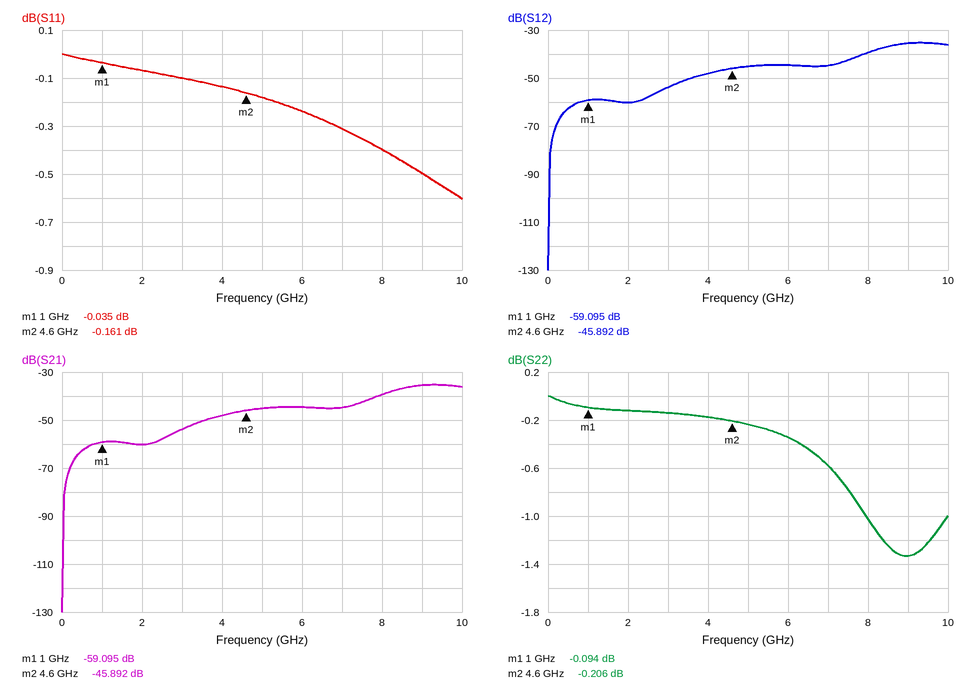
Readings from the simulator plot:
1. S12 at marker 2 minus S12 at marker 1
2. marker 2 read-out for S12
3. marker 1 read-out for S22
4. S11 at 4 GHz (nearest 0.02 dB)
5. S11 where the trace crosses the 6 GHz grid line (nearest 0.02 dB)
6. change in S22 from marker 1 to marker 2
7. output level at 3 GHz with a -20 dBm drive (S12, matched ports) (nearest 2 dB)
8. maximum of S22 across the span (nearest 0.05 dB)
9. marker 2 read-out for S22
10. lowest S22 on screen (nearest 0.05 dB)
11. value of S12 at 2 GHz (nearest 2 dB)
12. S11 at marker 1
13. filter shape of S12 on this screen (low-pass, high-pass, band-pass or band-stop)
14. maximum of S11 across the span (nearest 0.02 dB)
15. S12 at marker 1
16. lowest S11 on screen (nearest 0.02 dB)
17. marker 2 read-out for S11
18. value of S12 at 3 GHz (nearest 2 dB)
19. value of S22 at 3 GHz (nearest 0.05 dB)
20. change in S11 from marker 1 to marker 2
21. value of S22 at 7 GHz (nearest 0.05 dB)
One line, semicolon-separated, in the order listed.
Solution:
13.203 dB; -45.892 dB; -0.094 dB; -0.14 dB; -0.24 dB; -0.112 dB; -74 dBm; 0.00 dB; -0.206 dB; -1.35 dB; -60 dB; -0.035 dB; high-pass; 0.00 dB; -59.095 dB; -0.60 dB; -0.161 dB; -54 dB; -0.15 dB; -0.126 dB; -0.60 dB
